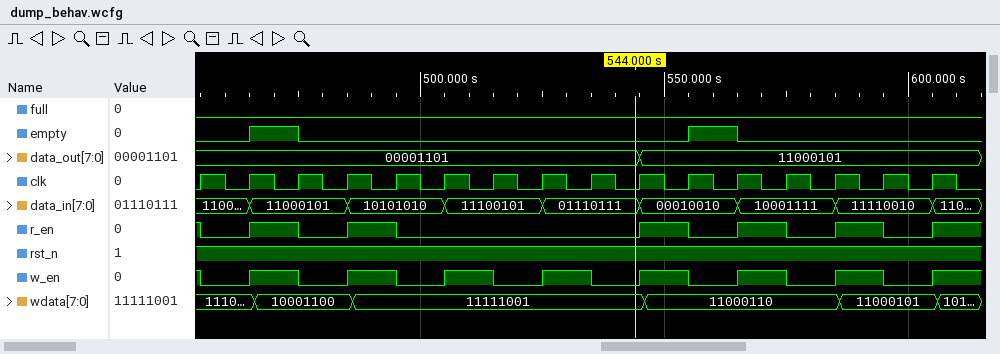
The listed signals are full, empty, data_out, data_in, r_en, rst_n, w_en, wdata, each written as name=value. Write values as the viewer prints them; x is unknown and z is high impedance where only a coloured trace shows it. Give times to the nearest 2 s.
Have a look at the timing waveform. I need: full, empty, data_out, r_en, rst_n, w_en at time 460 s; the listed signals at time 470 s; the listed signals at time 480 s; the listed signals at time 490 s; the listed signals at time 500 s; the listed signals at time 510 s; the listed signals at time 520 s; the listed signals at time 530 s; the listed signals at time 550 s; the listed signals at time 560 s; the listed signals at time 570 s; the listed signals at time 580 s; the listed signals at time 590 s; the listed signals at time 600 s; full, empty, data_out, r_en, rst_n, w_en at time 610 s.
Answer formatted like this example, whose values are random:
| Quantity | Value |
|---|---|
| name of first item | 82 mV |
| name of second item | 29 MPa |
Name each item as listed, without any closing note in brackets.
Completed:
| Quantity | Value |
|---|---|
| full, empty, data_out, r_en, rst_n, w_en at time 460 s | full=0, empty=0, data_out=00001101, r_en=0, rst_n=1, w_en=0 |
| the listed signals at time 470 s | full=0, empty=1, data_out=00001101, data_in=11000101, r_en=1, rst_n=1, w_en=1, wdata=10001100 |
| the listed signals at time 480 s | full=0, empty=0, data_out=00001101, data_in=11000101, r_en=0, rst_n=1, w_en=0, wdata=10001100 |
| the listed signals at time 490 s | full=0, empty=0, data_out=00001101, data_in=10101010, r_en=1, rst_n=1, w_en=1, wdata=11111001 |
| the listed signals at time 500 s | full=0, empty=0, data_out=00001101, data_in=10101010, r_en=0, rst_n=1, w_en=0, wdata=11111001 |
| the listed signals at time 510 s | full=0, empty=0, data_out=00001101, data_in=11100101, r_en=0, rst_n=1, w_en=1, wdata=11111001 |
| the listed signals at time 520 s | full=0, empty=0, data_out=00001101, data_in=11100101, r_en=0, rst_n=1, w_en=0, wdata=11111001 |
| the listed signals at time 530 s | full=0, empty=0, data_out=00001101, data_in=01110111, r_en=0, rst_n=1, w_en=1, wdata=11111001 |
| the listed signals at time 550 s | full=0, empty=0, data_out=11000101, data_in=00010010, r_en=1, rst_n=1, w_en=1, wdata=11000110 |
| the listed signals at time 560 s | full=0, empty=1, data_out=11000101, data_in=00010010, r_en=0, rst_n=1, w_en=0, wdata=11000110 |
| the listed signals at time 570 s | full=0, empty=0, data_out=11000101, data_in=10001111, r_en=1, rst_n=1, w_en=1, wdata=11000110 |
| the listed signals at time 580 s | full=0, empty=0, data_out=11000101, data_in=10001111, r_en=0, rst_n=1, w_en=0, wdata=11000110 |
| the listed signals at time 590 s | full=0, empty=0, data_out=11000101, data_in=11110010, r_en=1, rst_n=1, w_en=1, wdata=11000101 |
| the listed signals at time 600 s | full=0, empty=0, data_out=11000101, data_in=11110010, r_en=0, rst_n=1, w_en=0, wdata=11000101 |
| full, empty, data_out, r_en, rst_n, w_en at time 610 s | full=0, empty=0, data_out=11000101, r_en=1, rst_n=1, w_en=1 |
